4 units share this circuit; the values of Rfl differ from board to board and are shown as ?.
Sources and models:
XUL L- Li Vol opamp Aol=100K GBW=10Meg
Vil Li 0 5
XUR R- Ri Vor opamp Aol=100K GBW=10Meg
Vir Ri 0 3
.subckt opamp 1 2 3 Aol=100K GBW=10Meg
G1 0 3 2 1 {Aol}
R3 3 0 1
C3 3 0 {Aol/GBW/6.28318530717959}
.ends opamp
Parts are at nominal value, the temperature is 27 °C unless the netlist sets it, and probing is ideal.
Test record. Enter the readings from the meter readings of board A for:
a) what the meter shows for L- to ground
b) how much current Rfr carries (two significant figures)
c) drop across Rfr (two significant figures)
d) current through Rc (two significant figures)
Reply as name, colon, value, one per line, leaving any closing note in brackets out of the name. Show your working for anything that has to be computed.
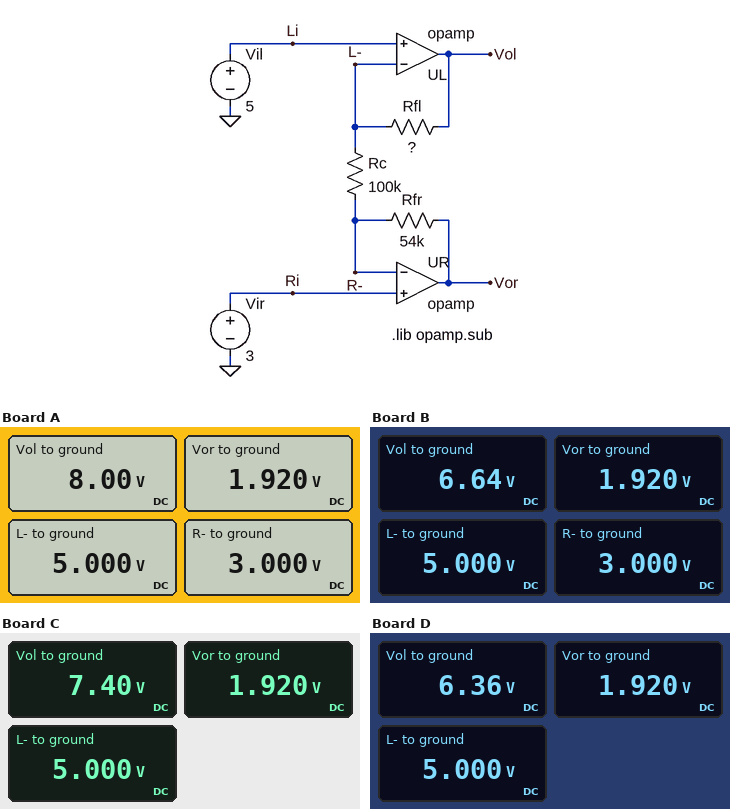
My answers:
what the meter shows for L- to ground: 5.000 V
how much current Rfr carries: (3 V - 1.92 V) / 54 kΩ = 20 µA
drop across Rfr: 3 V - 1.92 V = 1.1 V
current through Rc: (5 V - 3 V) / 100 kΩ = 20 µA
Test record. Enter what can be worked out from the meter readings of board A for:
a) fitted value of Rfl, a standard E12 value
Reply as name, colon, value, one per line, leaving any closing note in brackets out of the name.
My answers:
fitted value of Rfl, a standard E12 value: 150 kΩ
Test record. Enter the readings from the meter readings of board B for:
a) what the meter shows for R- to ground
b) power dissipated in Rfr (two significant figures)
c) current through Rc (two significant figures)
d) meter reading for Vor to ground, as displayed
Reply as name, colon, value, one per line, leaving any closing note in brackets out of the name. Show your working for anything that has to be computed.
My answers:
what the meter shows for R- to ground: 3.000 V
power dissipated in Rfr: (3 V - 1.92 V)^2 / 54 kΩ = 22 µW
current through Rc: (5 V - 3 V) / 100 kΩ = 20 µA
meter reading for Vor to ground, as displayed: 1.920 V
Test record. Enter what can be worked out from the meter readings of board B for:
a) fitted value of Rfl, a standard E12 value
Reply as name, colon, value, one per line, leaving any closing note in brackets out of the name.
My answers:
fitted value of Rfl, a standard E12 value: 82 kΩ
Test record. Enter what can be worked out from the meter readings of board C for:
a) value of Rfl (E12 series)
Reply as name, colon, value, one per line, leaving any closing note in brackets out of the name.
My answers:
value of Rfl: 120 kΩ
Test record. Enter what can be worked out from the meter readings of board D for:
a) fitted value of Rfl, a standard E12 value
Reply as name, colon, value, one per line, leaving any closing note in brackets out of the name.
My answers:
fitted value of Rfl, a standard E12 value: 68 kΩ
